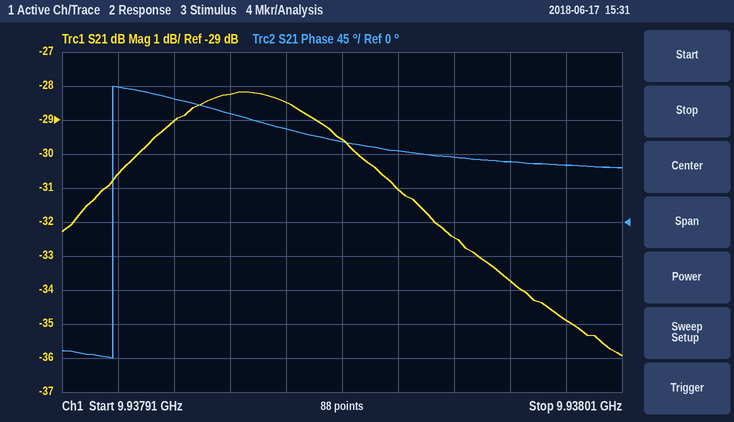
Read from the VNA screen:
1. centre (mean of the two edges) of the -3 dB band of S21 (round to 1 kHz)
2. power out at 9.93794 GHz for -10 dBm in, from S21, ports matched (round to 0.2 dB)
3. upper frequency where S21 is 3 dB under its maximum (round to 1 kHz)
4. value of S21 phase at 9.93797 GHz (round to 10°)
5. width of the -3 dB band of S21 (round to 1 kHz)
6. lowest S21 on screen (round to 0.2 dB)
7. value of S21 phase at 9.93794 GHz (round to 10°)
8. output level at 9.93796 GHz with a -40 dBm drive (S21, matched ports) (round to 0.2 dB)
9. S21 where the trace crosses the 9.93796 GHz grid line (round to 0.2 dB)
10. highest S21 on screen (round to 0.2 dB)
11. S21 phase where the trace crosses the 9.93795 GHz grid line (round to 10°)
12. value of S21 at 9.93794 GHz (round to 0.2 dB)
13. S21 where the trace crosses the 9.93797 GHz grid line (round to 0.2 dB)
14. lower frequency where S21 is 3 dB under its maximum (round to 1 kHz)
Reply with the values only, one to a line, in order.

9.937944 GHz
-38.2 dBm
9.937971 GHz
90°
54 kHz
-36.0 dB
140°
-69.6 dBm
-29.6 dB
-28.2 dB
120°
-28.2 dB
-31.0 dB
9.937917 GHz
